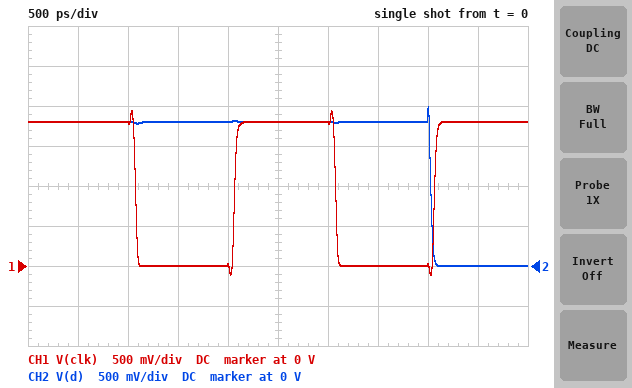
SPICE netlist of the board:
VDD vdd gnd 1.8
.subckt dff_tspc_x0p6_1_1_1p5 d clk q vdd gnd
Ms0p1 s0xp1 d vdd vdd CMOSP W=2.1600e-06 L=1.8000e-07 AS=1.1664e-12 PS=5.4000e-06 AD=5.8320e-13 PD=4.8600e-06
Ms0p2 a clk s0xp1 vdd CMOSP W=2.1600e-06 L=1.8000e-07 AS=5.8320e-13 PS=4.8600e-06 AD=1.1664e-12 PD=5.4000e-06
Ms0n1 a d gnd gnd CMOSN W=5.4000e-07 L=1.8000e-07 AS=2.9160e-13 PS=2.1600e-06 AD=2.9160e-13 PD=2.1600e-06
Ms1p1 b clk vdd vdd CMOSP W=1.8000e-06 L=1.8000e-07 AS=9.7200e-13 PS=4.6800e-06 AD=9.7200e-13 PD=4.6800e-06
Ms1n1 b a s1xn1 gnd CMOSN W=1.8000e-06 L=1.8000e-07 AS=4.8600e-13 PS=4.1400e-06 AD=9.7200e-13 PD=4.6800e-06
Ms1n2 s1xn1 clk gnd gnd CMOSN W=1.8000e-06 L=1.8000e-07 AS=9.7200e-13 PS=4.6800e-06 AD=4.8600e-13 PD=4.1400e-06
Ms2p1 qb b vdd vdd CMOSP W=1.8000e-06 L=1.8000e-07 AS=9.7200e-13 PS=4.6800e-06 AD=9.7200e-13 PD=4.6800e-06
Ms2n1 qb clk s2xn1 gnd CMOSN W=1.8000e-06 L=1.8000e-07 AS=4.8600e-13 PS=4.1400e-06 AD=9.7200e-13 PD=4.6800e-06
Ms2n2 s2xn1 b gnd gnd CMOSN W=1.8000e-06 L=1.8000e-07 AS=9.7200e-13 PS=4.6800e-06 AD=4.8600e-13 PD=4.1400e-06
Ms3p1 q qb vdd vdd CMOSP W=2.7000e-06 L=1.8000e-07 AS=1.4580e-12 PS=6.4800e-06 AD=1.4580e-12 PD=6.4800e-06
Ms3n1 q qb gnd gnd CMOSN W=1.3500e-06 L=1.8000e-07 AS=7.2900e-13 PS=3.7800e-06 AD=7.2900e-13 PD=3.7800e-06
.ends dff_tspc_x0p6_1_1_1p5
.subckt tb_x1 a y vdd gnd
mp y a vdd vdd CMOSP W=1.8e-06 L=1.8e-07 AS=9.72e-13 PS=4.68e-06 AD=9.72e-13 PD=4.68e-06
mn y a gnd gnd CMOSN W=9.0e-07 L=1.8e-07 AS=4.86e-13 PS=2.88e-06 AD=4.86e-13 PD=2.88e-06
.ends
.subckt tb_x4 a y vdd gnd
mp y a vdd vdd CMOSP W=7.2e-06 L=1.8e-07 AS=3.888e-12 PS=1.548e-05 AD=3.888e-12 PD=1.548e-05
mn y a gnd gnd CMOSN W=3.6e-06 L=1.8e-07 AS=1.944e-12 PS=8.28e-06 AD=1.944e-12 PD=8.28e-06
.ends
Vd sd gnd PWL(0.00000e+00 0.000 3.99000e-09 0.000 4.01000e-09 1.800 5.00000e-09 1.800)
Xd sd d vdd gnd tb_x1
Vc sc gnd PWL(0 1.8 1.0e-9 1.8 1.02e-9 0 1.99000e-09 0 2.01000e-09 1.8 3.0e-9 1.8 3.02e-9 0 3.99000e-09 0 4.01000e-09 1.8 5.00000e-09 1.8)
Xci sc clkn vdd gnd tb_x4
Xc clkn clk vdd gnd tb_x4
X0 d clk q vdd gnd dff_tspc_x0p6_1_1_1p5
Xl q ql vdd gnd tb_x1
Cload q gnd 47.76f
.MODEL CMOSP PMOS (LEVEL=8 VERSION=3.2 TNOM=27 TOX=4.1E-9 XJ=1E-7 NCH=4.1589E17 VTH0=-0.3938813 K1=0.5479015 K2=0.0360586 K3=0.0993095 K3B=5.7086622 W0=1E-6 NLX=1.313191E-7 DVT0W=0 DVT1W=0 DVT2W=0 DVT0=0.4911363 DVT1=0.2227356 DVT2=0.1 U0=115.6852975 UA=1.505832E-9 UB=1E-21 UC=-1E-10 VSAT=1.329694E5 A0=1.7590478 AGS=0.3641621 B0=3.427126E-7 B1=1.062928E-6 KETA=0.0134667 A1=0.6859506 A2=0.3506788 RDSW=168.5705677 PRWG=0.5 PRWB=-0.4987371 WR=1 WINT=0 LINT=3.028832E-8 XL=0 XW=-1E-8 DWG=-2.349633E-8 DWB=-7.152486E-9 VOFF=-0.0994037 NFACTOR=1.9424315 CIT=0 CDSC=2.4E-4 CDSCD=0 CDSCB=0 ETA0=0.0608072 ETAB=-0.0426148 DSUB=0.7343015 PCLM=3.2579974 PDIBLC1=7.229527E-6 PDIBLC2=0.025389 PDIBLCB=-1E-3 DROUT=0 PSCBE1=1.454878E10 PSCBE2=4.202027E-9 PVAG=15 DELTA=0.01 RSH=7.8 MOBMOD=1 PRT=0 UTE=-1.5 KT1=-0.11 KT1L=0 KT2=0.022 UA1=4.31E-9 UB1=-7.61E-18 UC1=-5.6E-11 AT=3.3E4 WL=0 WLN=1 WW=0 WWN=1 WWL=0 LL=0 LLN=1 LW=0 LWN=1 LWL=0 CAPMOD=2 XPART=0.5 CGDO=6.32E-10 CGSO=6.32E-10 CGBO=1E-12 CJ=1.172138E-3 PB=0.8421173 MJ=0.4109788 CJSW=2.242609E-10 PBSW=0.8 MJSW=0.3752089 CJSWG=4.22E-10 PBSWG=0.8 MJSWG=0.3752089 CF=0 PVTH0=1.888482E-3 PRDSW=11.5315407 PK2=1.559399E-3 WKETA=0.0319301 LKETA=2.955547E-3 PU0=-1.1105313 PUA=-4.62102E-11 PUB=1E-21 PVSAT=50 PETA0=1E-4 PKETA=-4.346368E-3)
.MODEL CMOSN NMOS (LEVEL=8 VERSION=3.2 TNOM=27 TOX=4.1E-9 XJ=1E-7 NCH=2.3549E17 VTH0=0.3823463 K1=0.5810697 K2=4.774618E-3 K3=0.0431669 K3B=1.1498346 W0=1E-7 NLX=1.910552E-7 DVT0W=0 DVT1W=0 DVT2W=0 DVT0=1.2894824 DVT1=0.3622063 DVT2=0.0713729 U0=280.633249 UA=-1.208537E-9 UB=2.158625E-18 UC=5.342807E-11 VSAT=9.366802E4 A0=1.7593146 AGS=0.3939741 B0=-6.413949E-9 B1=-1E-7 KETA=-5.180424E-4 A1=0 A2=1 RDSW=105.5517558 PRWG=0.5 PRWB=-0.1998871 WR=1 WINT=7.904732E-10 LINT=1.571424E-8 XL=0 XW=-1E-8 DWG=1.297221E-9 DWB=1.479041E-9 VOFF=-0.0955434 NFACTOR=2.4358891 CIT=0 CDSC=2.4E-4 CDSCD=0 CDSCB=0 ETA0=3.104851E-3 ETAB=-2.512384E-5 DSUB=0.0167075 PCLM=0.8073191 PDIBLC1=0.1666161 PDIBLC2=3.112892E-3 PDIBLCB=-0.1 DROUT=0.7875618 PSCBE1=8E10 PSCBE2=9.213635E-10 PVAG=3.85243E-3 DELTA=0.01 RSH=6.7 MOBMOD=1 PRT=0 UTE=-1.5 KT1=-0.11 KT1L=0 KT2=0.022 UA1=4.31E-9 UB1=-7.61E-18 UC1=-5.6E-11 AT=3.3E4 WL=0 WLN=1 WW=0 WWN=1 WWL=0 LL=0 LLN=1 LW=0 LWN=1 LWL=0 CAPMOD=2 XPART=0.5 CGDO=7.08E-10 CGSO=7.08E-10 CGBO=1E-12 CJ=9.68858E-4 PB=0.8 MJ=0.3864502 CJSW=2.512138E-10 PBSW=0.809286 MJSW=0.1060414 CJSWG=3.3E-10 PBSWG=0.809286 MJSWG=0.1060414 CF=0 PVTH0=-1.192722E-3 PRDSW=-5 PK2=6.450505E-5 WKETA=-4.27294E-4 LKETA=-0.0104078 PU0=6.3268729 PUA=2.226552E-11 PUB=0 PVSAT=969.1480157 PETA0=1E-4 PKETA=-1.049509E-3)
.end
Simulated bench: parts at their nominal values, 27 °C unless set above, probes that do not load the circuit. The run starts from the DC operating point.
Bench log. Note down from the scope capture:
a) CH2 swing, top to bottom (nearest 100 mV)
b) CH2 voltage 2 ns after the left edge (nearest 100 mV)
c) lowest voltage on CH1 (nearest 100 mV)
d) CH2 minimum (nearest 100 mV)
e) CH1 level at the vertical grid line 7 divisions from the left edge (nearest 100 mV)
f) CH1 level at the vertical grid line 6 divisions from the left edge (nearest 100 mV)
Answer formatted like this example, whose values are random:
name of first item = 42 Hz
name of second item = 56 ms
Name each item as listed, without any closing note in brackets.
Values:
CH2 swing, top to bottom = 2.0 V
CH2 voltage 2 ns after the left edge = 1.8 V
lowest voltage on CH1 = -100 mV
CH2 minimum = 0 V
CH1 level at the vertical grid line 7 divisions from the left edge = 0 V
CH1 level at the vertical grid line 6 divisions from the left edge = 1.8 V
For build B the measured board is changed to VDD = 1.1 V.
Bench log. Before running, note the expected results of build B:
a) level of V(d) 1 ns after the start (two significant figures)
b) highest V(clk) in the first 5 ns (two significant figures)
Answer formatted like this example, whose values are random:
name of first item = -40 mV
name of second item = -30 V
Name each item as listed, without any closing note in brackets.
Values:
level of V(d) 1 ns after the start = 1.1 V
highest V(clk) in the first 5 ns = 1.2 V
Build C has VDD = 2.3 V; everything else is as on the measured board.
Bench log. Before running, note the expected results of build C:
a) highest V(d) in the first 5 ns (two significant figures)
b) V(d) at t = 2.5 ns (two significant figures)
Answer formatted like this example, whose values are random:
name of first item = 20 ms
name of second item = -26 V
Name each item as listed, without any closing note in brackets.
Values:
highest V(d) in the first 5 ns = 2.5 V
V(d) at t = 2.5 ns = 2.3 V
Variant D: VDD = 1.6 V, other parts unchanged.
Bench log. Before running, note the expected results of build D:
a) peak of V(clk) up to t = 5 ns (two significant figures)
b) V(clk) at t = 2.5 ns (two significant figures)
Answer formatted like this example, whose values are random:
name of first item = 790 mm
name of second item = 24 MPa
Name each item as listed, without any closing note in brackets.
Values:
peak of V(clk) up to t = 5 ns = 1.7 V
V(clk) at t = 2.5 ns = 1.6 V
